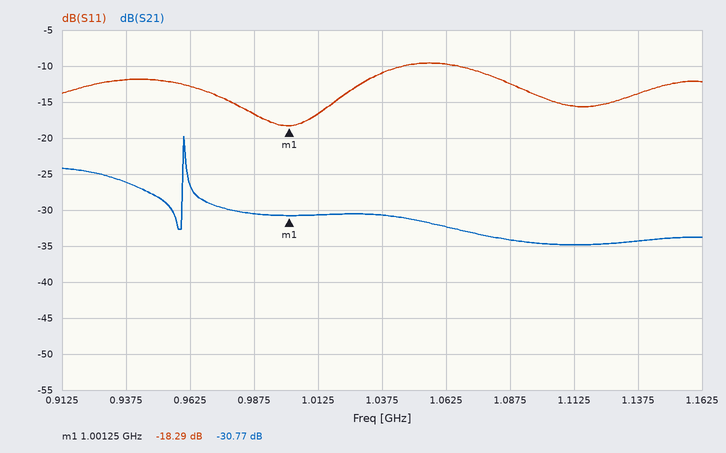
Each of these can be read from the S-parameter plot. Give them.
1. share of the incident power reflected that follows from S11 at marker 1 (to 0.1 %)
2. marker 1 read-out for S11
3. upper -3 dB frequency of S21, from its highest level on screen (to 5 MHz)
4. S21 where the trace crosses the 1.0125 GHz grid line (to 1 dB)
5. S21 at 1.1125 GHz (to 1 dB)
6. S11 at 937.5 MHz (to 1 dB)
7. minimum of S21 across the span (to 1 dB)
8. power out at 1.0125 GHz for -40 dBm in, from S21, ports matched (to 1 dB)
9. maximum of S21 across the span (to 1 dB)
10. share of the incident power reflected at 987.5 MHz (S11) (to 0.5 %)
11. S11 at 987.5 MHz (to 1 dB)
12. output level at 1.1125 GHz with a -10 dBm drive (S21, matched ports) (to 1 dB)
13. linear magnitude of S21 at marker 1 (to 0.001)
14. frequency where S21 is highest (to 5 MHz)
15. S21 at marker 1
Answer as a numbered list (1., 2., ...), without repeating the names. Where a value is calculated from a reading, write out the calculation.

1. 10^(-18.29/10) ≈ 1.5 %
2. -18.29 dB
3. 960 MHz
4. -31 dB
5. -35 dB
6. -12 dB
7. -35 dB
8. -40 dBm + (-31 dB) = -71 dBm
9. -20 dB
10. 10^(-17/10) ≈ 2.0 %
11. -17 dB
12. -10 dBm + (-35 dB) = -45 dBm
13. 10^(-30.77/20) ≈ 0.029
14. 960 MHz
15. -30.77 dB
